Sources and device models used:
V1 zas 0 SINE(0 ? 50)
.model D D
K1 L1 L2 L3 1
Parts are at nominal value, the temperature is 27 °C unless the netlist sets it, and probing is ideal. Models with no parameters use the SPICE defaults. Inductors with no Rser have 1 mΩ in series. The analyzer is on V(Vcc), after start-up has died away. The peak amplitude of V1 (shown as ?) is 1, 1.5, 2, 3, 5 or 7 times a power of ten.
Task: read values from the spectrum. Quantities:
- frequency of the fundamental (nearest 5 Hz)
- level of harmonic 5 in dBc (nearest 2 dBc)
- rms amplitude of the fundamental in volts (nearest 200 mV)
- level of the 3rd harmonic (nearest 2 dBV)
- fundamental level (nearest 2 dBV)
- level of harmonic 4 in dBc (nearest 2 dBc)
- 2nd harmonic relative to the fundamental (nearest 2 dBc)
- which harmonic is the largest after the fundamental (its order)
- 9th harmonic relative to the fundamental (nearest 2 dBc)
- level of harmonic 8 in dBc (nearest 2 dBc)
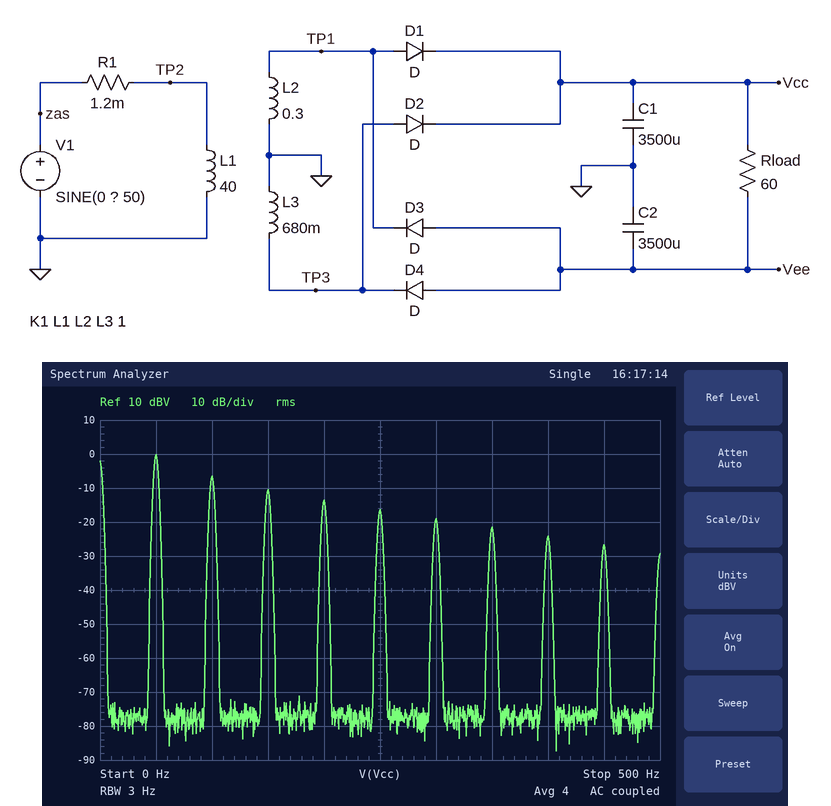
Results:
50 Hz
-16 dBc
1.0 V
-10 dBV
0 dBV
-14 dBc
-6 dBc
2
-26 dBc
-24 dBc
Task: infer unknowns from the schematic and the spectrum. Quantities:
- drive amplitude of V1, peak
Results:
200 V
